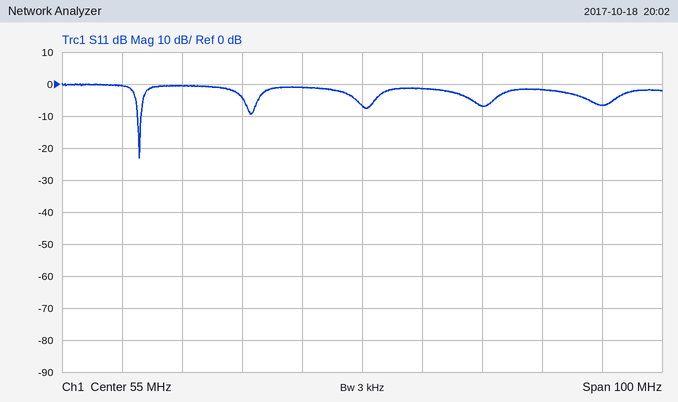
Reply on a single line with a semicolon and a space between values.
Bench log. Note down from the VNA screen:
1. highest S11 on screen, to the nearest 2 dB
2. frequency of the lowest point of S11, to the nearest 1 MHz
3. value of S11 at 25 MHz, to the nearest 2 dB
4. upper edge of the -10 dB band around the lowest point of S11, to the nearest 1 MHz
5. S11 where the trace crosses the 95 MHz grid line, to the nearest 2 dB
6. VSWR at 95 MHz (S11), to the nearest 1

0 dB; 18 MHz; 0 dB; 18 MHz; -6 dB; 3
